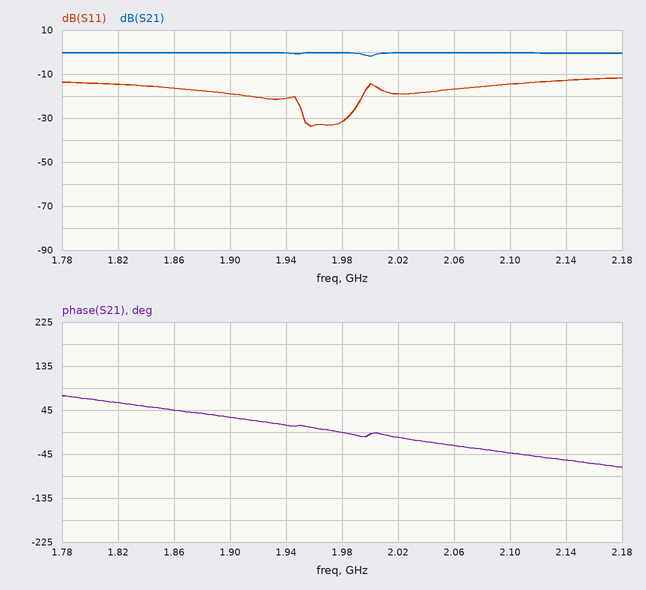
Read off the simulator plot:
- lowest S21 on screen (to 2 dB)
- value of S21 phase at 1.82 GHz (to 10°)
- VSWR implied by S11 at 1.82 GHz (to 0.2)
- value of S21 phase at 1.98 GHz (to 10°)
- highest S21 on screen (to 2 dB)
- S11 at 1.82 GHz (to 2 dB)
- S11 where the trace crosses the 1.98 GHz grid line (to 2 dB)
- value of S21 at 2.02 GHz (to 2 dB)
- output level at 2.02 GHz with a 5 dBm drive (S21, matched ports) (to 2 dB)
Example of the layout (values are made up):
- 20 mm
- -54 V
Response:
- -2 dB
- 60°
- 1.4
- 0°
- 0 dB
- -14 dB
- -32 dB
- 0 dB
- 4 dBm
